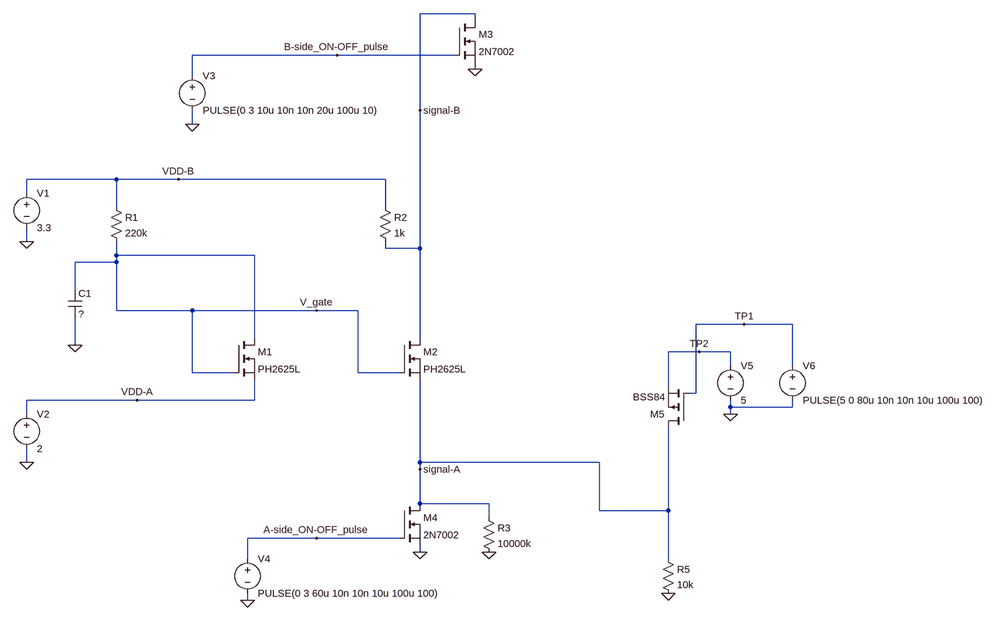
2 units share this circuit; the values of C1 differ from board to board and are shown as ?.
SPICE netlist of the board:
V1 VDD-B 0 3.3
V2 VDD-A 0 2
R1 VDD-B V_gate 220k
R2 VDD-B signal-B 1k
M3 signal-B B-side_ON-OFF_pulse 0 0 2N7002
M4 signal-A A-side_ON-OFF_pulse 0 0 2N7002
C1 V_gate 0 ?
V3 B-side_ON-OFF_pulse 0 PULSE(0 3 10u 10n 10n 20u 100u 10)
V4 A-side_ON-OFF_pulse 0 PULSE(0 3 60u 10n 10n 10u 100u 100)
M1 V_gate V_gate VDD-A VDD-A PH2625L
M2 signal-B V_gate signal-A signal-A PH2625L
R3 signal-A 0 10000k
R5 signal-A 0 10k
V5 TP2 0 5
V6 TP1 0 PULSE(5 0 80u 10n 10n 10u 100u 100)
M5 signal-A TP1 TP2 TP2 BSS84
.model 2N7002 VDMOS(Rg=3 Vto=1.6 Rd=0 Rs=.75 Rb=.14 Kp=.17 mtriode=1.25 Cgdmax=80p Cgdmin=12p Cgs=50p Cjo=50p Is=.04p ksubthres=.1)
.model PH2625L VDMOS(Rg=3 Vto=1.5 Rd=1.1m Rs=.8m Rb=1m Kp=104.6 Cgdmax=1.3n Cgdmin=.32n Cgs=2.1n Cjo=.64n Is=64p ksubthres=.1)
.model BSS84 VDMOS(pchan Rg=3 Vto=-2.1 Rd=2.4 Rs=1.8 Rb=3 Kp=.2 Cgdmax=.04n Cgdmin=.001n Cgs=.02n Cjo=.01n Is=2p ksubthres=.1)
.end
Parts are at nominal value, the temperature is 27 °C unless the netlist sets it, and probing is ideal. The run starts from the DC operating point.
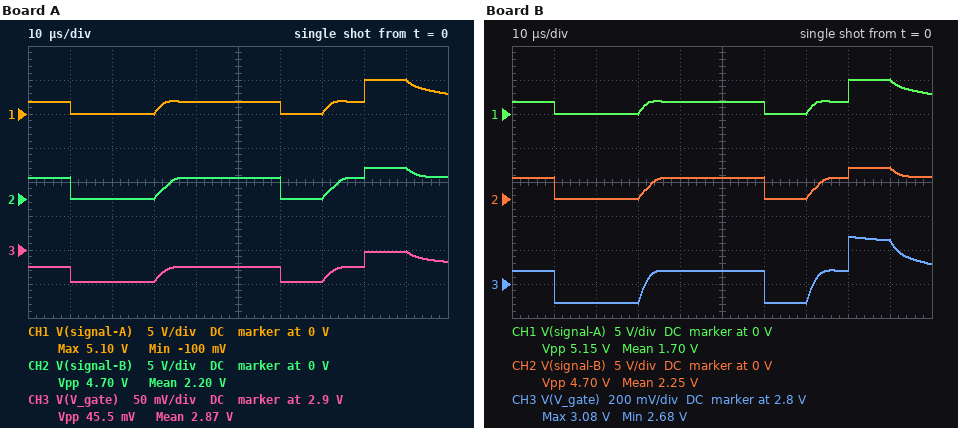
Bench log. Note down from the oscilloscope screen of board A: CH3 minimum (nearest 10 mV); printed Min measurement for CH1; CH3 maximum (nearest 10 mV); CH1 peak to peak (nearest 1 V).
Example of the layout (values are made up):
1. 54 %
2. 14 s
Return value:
1. 2.85 V
2. -100 mV
3. 2.90 V
4. 5 V
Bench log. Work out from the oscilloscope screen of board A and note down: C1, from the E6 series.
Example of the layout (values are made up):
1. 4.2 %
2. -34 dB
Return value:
1. 330 nF
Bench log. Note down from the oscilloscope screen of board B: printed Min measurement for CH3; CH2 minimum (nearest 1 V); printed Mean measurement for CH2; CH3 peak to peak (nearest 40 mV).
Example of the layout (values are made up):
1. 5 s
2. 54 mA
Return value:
1. 2.68 V
2. 0 V
3. 2.25 V
4. 400 mV
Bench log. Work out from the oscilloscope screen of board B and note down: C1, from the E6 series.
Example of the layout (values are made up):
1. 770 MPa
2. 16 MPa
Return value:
1. 33 nF
